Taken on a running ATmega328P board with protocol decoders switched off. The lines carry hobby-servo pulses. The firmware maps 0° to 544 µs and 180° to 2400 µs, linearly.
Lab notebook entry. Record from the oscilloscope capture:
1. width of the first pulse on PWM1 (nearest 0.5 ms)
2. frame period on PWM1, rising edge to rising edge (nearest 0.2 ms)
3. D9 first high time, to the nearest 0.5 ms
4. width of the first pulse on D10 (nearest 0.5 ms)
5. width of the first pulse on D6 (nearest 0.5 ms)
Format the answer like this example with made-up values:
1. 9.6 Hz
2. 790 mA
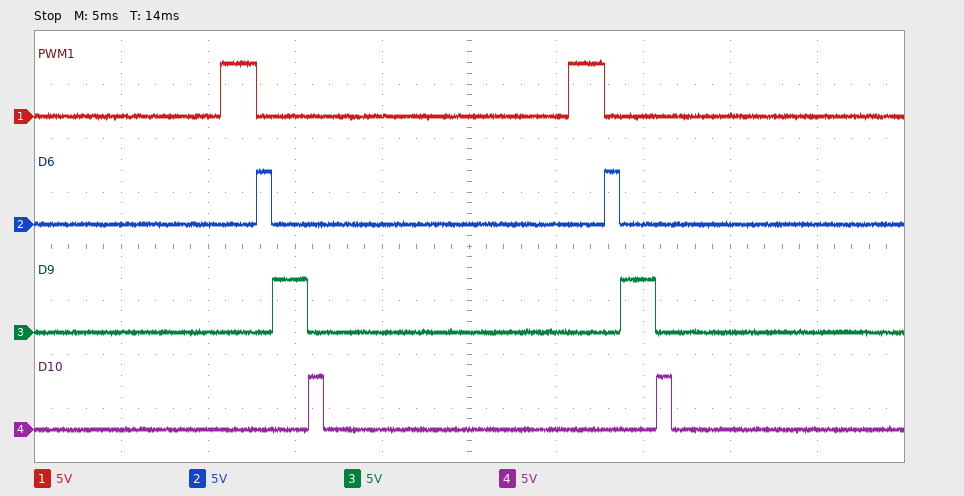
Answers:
1. 2.0 ms
2. 20.0 ms
3. 2.0 ms
4. 1.0 ms
5. 1.0 ms
